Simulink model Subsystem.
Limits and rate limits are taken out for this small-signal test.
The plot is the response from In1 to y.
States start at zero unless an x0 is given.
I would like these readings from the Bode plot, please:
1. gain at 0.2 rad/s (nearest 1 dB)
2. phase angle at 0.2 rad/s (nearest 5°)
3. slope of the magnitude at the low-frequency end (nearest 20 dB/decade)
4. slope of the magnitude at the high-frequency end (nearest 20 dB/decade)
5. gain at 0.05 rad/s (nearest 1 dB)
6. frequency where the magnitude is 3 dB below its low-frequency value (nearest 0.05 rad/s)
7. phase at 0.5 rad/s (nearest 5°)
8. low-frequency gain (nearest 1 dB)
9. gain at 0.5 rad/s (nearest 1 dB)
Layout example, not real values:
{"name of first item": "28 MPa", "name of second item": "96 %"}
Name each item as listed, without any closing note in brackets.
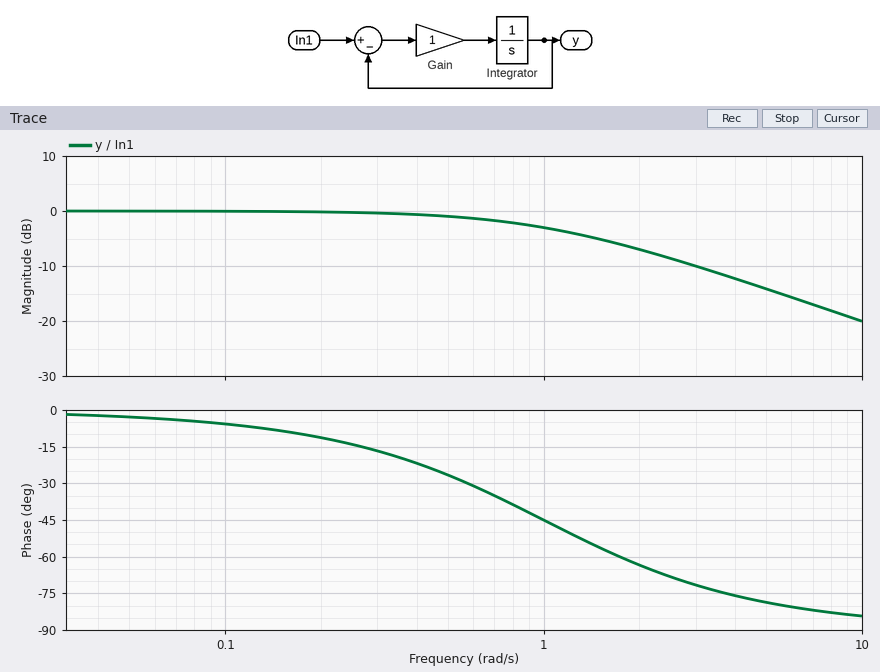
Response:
{"gain at 0.2 rad/s": "0 dB", "phase angle at 0.2 rad/s": "-10°", "slope of the magnitude at the low-frequency end": "0 dB/decade", "slope of the magnitude at the high-frequency end": "-20 dB/decade", "gain at 0.05 rad/s": "0 dB", "frequency where the magnitude is 3 dB below its low-frequency value": "1.00 rad/s", "phase at 0.5 rad/s": "-25°", "low-frequency gain": "0 dB", "gain at 0.5 rad/s": "-1 dB"}
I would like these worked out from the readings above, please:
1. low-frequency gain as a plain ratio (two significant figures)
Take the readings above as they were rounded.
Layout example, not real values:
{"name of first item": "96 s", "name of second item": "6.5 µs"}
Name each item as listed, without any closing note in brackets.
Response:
{"low-frequency gain as a plain ratio": "1.0"}
